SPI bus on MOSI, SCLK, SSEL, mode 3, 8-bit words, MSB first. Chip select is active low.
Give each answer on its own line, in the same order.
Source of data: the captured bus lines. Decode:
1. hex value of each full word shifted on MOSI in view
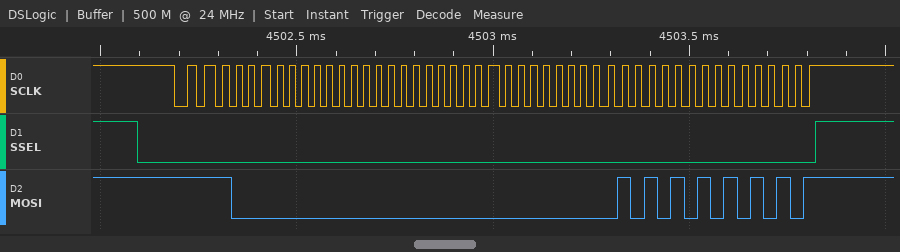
E0, 00, 00, 00, 55, 55
